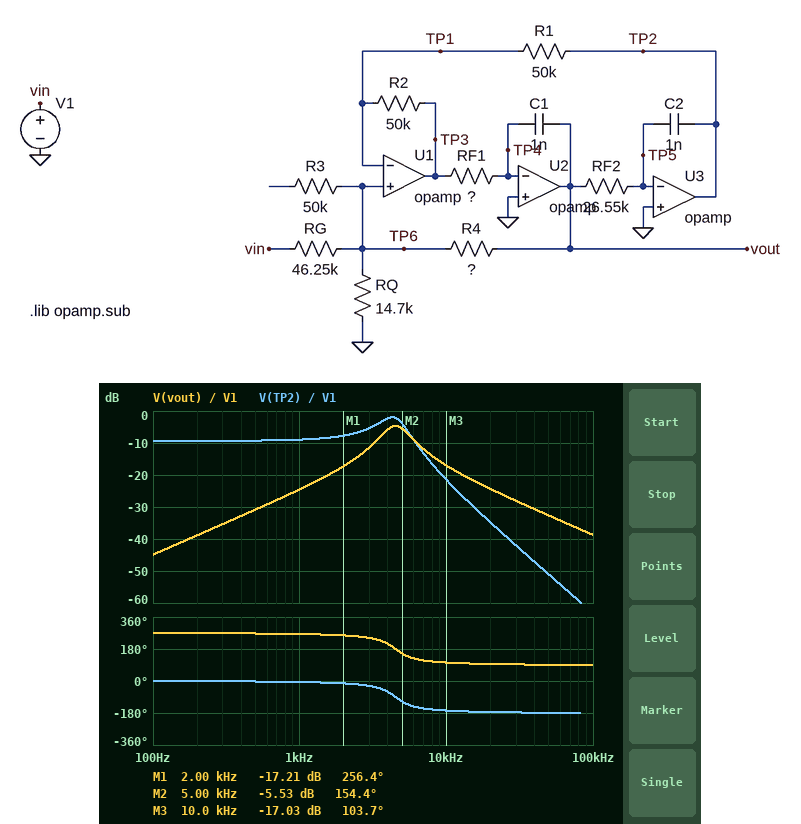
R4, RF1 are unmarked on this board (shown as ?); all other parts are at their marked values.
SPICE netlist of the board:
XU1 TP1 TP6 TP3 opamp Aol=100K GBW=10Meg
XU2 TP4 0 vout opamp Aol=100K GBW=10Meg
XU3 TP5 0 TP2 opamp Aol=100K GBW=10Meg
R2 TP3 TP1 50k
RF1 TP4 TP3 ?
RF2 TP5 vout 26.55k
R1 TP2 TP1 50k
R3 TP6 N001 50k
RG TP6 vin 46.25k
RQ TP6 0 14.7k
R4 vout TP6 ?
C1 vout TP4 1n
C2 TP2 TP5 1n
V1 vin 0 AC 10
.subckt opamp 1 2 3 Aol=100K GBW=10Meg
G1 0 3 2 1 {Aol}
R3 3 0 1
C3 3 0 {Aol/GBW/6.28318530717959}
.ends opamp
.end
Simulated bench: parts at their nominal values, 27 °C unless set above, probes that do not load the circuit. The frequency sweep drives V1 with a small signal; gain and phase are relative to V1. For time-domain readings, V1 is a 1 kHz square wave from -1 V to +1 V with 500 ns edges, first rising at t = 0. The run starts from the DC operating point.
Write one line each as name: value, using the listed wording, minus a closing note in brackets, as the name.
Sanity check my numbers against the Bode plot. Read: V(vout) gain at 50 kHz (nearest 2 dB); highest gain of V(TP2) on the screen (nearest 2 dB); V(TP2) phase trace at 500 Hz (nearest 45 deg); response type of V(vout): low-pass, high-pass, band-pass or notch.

V(vout) gain at 50 kHz: -32 dB
highest gain of V(TP2) on the screen: -2 dB
V(TP2) phase trace at 500 Hz: 0 deg
response type of V(vout): low-pass, high-pass, band-pass or notch: band-pass
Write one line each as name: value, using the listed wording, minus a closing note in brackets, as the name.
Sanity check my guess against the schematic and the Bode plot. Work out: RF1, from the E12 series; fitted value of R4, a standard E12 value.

RF1, from the E12 series: 47 kΩ
fitted value of R4, a standard E12 value: 27 kΩ
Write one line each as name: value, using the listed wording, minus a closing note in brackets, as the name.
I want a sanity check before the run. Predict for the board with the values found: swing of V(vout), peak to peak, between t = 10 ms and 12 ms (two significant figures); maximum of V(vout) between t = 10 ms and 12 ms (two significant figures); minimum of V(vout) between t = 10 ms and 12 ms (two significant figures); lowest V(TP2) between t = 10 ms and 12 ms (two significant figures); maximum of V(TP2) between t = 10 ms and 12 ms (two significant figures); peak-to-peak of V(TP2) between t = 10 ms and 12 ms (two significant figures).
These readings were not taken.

swing of V(vout), peak to peak, between t = 10 ms and 12 ms: 740 mV
maximum of V(vout) between t = 10 ms and 12 ms: 370 mV
minimum of V(vout) between t = 10 ms and 12 ms: -370 mV
lowest V(TP2) between t = 10 ms and 12 ms: -670 mV
maximum of V(TP2) between t = 10 ms and 12 ms: 670 mV
peak-to-peak of V(TP2) between t = 10 ms and 12 ms: 1.3 V
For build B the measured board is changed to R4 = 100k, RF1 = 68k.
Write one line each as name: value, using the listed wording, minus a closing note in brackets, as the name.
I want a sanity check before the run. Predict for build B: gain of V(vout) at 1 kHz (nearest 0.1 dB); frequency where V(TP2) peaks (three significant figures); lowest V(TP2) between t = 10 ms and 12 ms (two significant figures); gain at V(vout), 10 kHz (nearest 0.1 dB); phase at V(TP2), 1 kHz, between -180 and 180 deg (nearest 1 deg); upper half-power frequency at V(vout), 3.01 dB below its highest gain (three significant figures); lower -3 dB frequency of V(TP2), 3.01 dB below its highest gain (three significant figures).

gain of V(vout) at 1 kHz: -22.2 dB
frequency where V(TP2) peaks: 3.73 kHz
lowest V(TP2) between t = 10 ms and 12 ms: -960 mV
gain at V(vout), 10 kHz: -18.6 dB
phase at V(TP2), 1 kHz, between -180 and 180 deg: -2 deg
upper half-power frequency at V(vout), 3.01 dB below its highest gain: 3.98 kHz
lower -3 dB frequency of V(TP2), 3.01 dB below its highest gain: 3.49 kHz
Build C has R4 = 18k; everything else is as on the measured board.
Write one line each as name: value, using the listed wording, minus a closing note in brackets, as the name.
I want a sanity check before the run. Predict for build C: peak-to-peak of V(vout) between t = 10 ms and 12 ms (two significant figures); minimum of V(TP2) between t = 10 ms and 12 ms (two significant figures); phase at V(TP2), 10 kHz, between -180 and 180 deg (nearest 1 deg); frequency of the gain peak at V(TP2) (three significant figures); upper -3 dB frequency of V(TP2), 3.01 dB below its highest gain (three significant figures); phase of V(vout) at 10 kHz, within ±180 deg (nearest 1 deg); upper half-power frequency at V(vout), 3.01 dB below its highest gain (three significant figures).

peak-to-peak of V(vout) between t = 10 ms and 12 ms: 600 mV
minimum of V(TP2) between t = 10 ms and 12 ms: -530 mV
phase at V(TP2), 10 kHz, between -180 and 180 deg: -162 deg
frequency of the gain peak at V(TP2): 4.12 kHz
upper -3 dB frequency of V(TP2), 3.01 dB below its highest gain: 5.30 kHz
phase of V(vout) at 10 kHz, within ±180 deg: 108 deg
upper half-power frequency at V(vout), 3.01 dB below its highest gain: 5.98 kHz
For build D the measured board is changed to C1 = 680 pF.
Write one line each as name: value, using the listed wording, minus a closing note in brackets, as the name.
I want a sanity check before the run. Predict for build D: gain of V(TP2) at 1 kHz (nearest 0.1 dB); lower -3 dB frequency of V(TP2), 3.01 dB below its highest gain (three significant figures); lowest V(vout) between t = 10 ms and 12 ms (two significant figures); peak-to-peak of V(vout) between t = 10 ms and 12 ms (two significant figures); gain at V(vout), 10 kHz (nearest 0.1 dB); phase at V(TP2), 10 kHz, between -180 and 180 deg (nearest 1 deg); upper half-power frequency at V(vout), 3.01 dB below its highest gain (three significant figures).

gain of V(TP2) at 1 kHz: -9.1 dB
lower -3 dB frequency of V(TP2), 3.01 dB below its highest gain: 3.22 kHz
lowest V(vout) between t = 10 ms and 12 ms: -440 mV
peak-to-peak of V(vout) between t = 10 ms and 12 ms: 880 mV
gain at V(vout), 10 kHz: -13.0 dB
phase at V(TP2), 10 kHz, between -180 and 180 deg: -158 deg
upper half-power frequency at V(vout), 3.01 dB below its highest gain: 7.10 kHz
